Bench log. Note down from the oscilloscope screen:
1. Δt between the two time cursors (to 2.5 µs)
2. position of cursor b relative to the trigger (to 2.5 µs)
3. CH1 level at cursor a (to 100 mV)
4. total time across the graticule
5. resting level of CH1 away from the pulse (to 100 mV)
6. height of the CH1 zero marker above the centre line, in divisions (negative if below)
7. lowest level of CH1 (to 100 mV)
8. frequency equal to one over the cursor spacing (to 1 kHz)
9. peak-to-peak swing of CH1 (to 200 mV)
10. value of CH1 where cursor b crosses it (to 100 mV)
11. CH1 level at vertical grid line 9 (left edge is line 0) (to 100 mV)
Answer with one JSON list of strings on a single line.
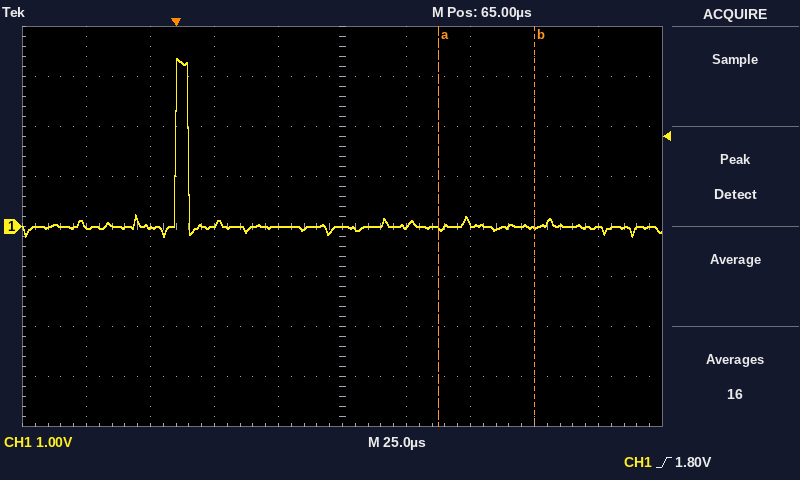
["37.5 µs", "+140.0 µs", "0.0 V", "250 µs", "0.0 V", "0.0 div", "-200 mV", "27 kHz", "3.6 V", "0.0 V", "0.0 V"]
